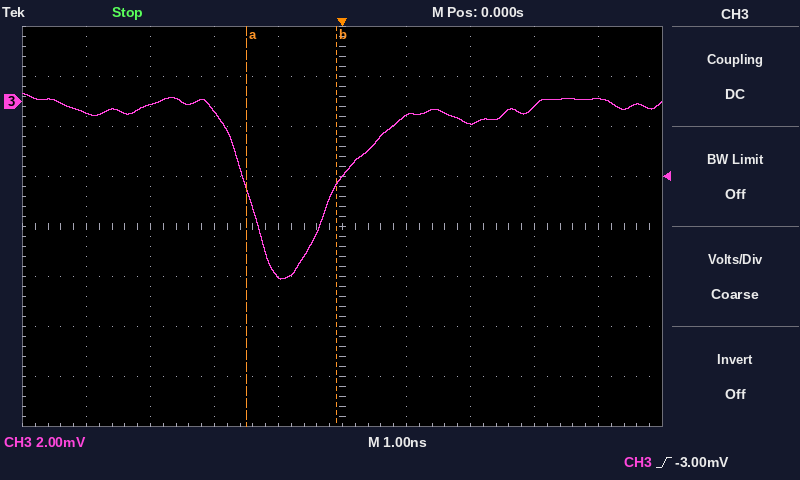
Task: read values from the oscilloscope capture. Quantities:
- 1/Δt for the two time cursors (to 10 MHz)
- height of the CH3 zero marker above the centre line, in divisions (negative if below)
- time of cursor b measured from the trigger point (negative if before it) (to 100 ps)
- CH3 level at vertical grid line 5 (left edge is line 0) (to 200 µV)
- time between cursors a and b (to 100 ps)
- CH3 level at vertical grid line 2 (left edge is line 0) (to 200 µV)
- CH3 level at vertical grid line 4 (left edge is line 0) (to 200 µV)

710 MHz
+2.5 div
-100 ps
-3.0 mV
1.4 ns
-200 µV
-7.0 mV
